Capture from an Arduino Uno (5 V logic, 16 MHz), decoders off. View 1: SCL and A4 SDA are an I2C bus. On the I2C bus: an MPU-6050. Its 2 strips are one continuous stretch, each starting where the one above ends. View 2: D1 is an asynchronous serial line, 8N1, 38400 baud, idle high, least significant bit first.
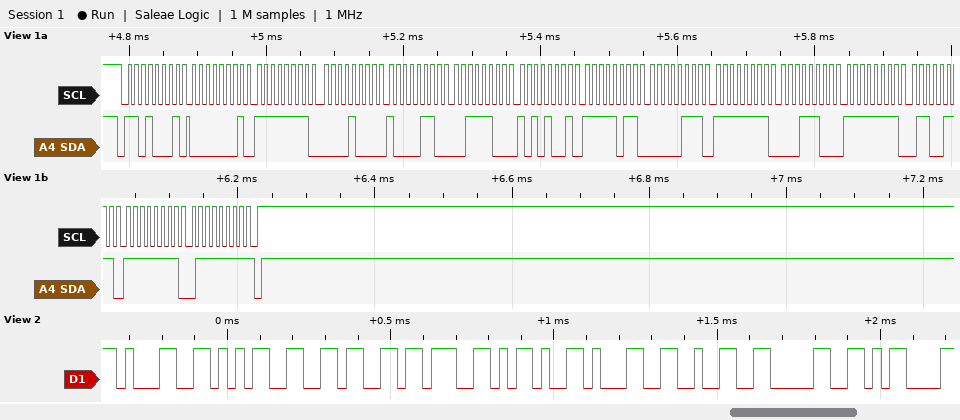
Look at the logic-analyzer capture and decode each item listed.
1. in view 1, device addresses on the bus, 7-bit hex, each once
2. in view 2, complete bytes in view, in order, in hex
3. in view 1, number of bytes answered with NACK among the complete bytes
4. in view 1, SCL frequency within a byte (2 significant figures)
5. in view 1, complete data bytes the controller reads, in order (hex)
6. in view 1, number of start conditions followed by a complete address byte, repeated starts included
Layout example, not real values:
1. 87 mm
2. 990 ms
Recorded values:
1. 0x68
2. 31 35 36 3B 2D 31 32 30 0D
3. 1
4. 100 kHz
5. 01 FF 08 86 3C A9 FB 07 FF 1C FF 67 FF 7F
6. 1
